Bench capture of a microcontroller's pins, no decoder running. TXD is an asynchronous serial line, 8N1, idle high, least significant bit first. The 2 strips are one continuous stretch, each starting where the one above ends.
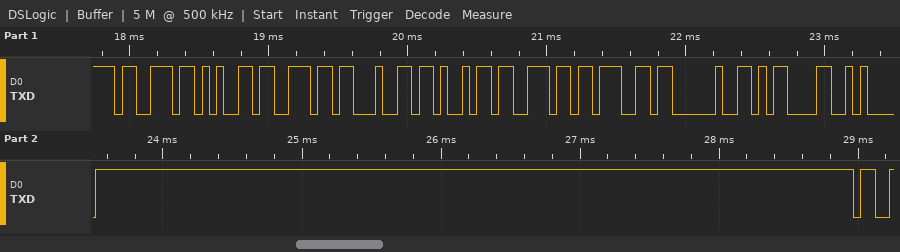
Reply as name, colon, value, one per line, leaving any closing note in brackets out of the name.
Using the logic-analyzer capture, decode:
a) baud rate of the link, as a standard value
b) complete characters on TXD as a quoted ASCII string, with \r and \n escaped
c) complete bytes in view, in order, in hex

baud rate of the link, as a standard value: 19200 baud
complete characters on TXD as a quoted ASCII string, with \r and \n escaped: "sending \r\n"
complete bytes in view, in order, in hex: 73 65 6E 64 69 6E 67 20 0D 0A
